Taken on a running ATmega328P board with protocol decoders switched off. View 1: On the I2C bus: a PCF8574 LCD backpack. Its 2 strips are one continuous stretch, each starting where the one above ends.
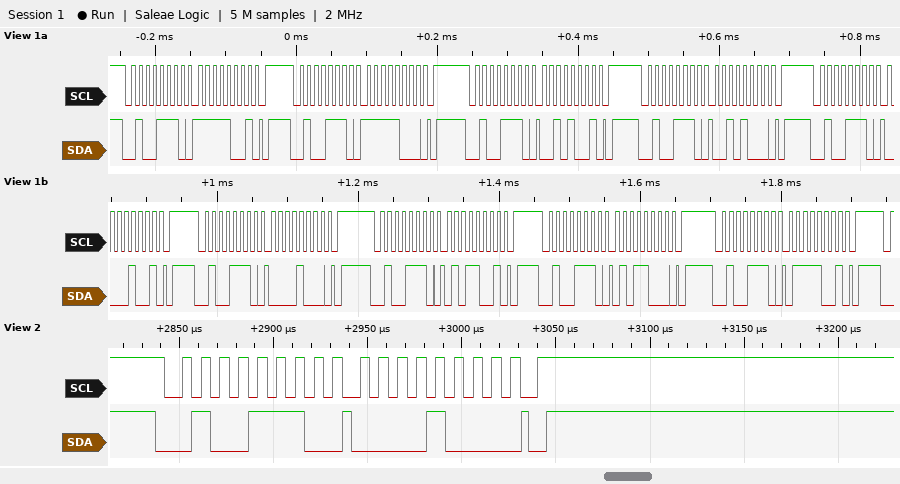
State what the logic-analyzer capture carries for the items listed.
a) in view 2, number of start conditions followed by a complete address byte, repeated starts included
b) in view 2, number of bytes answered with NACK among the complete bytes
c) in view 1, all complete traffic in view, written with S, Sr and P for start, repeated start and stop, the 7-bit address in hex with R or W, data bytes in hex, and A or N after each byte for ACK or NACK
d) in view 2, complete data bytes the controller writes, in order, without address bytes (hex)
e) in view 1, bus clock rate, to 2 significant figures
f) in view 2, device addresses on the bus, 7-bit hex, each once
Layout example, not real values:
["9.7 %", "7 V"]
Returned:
["1", "0", "S 27W A F9 A P S 27W A F8 A P S 27W A 29 A P S 27W A 28 A P S 27W A 09 A P S 27W A 08 A P S 27W A 59 A P S 27W A 58 A P S 27W A 79 A P", "08", "100 kHz", "0x27"]
